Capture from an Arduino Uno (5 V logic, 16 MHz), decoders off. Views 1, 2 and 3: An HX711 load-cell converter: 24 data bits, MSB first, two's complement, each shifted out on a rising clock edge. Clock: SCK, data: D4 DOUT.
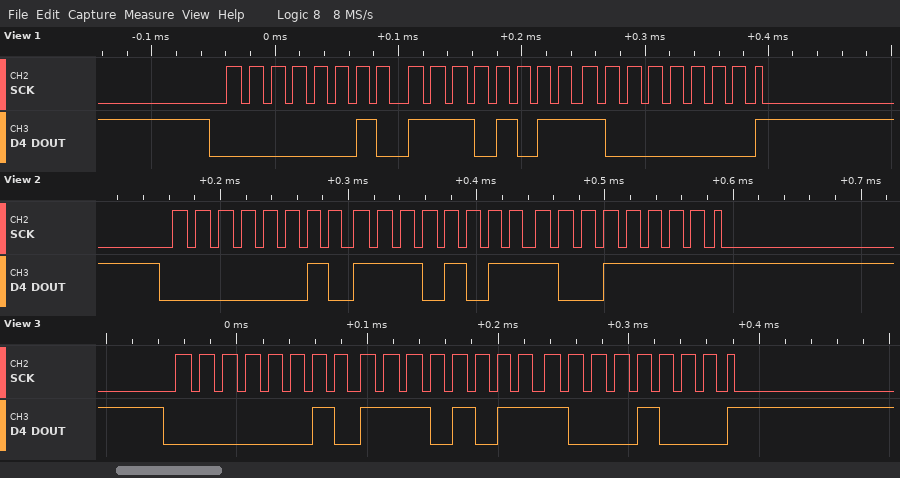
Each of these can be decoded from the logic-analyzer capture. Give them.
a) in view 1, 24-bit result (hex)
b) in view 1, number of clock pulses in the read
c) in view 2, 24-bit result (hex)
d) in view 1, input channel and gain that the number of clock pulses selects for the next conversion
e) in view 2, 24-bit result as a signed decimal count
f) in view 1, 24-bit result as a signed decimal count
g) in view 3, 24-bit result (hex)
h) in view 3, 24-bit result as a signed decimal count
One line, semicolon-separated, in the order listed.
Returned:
0x02EB80; 25; 0x02EB9F; channel A, gain 128; 191391; 191360; 0x02EB88; 191368
